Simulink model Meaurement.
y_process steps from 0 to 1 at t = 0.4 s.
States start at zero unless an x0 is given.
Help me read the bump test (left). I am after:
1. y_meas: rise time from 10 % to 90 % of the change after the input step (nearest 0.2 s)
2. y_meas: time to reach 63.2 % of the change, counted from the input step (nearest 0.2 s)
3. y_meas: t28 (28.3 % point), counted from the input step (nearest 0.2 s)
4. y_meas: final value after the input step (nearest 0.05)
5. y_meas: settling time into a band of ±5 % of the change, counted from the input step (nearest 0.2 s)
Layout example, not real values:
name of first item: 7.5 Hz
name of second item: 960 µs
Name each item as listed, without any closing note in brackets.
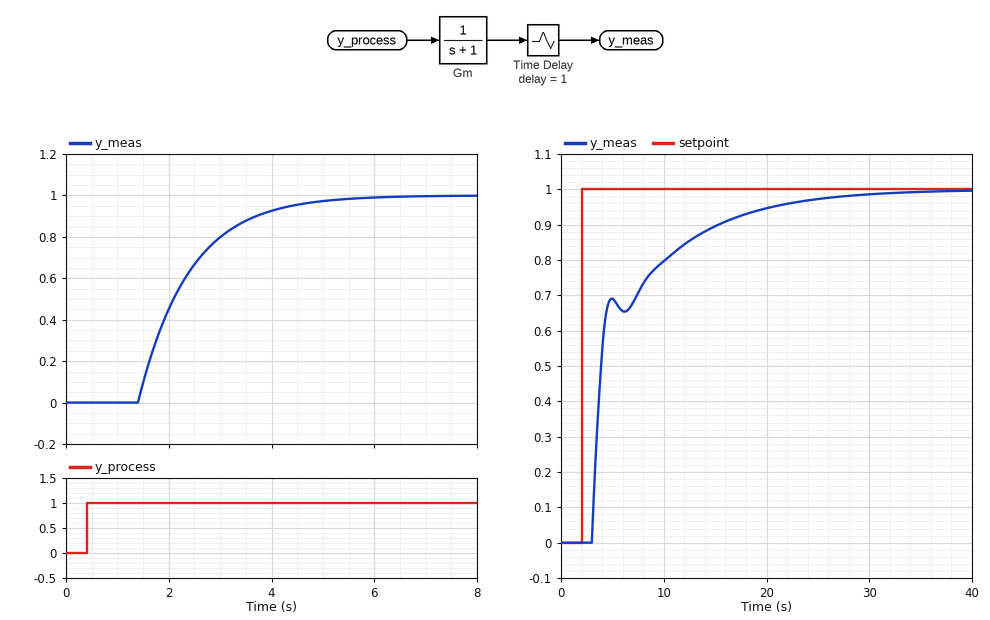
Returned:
y_meas: rise time from 10 % to 90 % of the change after the input step: 2.2 s
y_meas: time to reach 63.2 % of the change, counted from the input step: 2.0 s
y_meas: t28 (28.3 % point), counted from the input step: 1.4 s
y_meas: final value after the input step: 1.00
y_meas: settling time into a band of ±5 % of the change, counted from the input step: 4.0 s
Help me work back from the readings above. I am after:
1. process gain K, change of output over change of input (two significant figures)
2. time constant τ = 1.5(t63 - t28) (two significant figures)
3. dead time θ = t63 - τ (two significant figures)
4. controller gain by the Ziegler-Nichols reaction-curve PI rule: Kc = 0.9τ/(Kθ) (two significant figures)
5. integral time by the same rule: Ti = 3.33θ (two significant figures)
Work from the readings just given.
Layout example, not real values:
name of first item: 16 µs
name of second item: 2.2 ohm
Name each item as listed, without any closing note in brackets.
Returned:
process gain K, change of output over change of input: 1.0
time constant τ = 1.5(t63 - t28): 0.90 s
dead time θ = t63 - τ: 1.1 s
controller gain by the Ziegler-Nichols reaction-curve PI rule: Kc = 0.9τ/(Kθ): 0.74
integral time by the same rule: Ti = 3.33θ: 3.7 s
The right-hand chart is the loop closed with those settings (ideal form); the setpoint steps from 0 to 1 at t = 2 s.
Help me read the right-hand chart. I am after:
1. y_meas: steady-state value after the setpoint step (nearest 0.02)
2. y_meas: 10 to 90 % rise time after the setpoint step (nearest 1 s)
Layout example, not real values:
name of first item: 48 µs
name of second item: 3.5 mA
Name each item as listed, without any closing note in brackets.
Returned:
y_meas: steady-state value after the setpoint step: 1.00
y_meas: 10 to 90 % rise time after the setpoint step: 12 s
